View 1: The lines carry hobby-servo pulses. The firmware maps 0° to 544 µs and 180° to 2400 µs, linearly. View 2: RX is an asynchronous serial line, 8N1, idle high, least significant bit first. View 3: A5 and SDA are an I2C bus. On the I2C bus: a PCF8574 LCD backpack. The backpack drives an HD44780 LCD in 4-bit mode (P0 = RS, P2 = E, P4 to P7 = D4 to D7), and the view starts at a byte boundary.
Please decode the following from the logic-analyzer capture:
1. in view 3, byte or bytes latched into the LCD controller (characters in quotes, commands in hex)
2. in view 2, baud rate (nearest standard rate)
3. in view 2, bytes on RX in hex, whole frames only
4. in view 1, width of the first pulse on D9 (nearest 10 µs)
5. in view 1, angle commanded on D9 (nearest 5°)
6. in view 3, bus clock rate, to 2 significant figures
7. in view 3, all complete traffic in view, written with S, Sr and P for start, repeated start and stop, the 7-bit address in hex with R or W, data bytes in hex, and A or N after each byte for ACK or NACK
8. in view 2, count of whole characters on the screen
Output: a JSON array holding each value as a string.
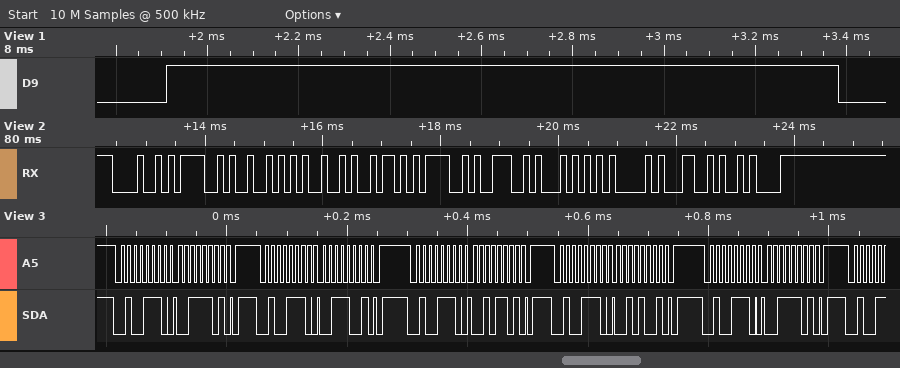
["'2'", "9600 baud", "48 4F 52 49 5A 4F 4E 54 41 4C 0A", "1470 µs", "90°", "100 kHz", "S 27W A 3D A P S 27W A 39 A P S 27W A 2D A P S 27W A 29 A P S 27W A 3D A P", "11"]
